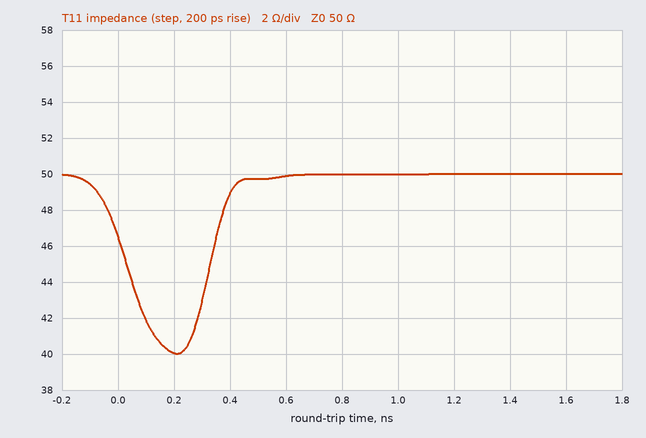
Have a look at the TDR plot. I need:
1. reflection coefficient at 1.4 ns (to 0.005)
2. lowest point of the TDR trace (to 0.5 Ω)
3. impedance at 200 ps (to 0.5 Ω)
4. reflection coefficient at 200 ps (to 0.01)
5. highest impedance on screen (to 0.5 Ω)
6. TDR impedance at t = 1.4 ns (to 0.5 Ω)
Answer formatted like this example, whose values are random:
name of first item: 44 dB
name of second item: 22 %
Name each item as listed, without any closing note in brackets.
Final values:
reflection coefficient at 1.4 ns: 0.000
lowest point of the TDR trace: 40.0 Ω
impedance at 200 ps: 40.0 Ω
reflection coefficient at 200 ps: -0.11
highest impedance on screen: 50.0 Ω
TDR impedance at t = 1.4 ns: 50.0 Ω
